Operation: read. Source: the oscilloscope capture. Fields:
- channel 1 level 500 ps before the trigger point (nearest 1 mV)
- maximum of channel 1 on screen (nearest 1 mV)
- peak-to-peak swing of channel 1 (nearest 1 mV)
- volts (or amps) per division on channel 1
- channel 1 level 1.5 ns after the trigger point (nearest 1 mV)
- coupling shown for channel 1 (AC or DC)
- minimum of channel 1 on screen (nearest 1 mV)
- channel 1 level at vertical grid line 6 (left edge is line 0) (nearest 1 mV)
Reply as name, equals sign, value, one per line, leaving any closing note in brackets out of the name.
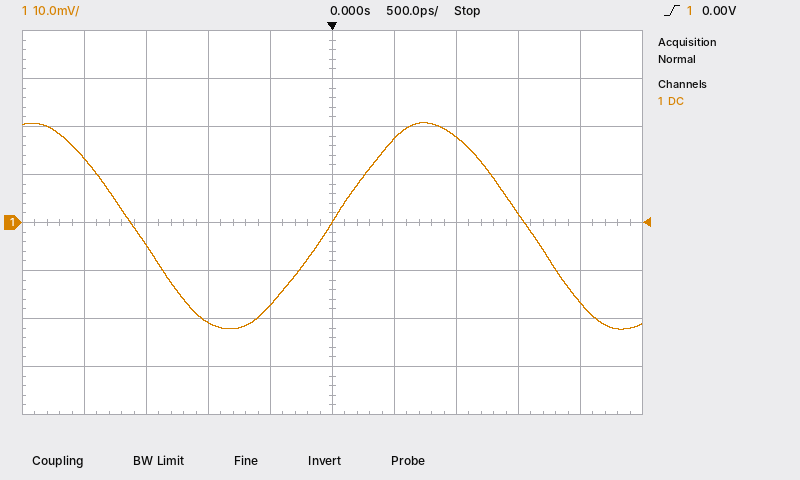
channel 1 level 500 ps before the trigger point = -17 mV
maximum of channel 1 on screen = 21 mV
peak-to-peak swing of channel 1 = 43 mV
volts (or amps) per division on channel 1 = 10 mV
channel 1 level 1.5 ns after the trigger point = 2 mV
coupling shown for channel 1 = DC
minimum of channel 1 on screen = -22 mV
channel 1 level at vertical grid line 6 (left edge is line 0) = 17 mV
